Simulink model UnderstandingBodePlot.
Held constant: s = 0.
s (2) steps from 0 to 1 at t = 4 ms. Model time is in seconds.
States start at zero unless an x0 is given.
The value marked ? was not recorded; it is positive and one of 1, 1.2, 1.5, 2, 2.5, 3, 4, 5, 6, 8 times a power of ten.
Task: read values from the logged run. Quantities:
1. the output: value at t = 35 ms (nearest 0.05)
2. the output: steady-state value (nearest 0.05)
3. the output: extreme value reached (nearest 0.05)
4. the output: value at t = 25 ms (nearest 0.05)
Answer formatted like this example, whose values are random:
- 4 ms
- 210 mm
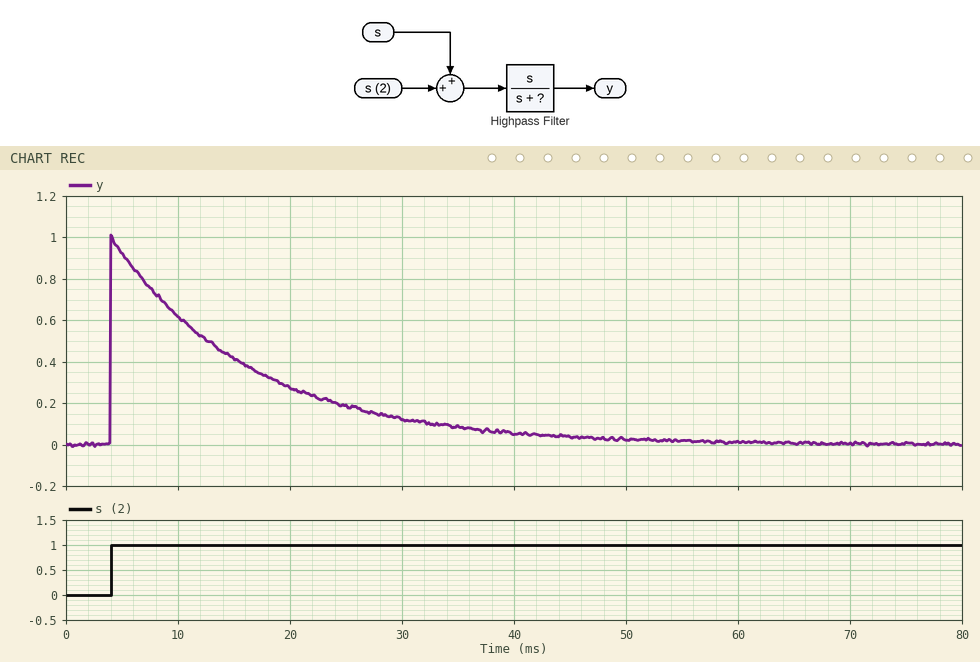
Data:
- 0.10
- 0.00
- 1.00
- 0.20
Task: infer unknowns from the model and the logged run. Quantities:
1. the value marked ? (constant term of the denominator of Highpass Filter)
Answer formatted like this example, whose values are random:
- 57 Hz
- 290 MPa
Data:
- 80
